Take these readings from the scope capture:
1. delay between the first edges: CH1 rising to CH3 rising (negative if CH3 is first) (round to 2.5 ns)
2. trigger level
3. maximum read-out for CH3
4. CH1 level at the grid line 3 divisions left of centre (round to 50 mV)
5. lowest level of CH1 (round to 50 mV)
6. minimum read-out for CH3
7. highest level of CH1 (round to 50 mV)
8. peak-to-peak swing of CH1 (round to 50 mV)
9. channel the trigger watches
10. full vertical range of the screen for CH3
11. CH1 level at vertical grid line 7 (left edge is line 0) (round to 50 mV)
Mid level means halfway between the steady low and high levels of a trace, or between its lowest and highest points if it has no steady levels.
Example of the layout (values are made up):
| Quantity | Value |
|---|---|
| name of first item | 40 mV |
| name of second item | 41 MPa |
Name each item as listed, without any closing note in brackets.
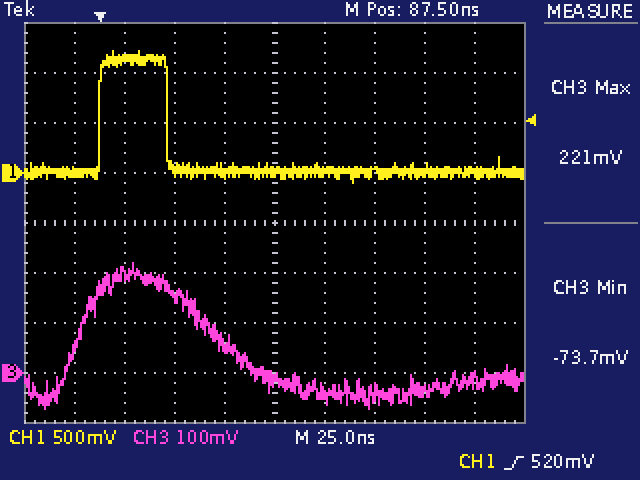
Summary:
| Quantity | Value |
|---|---|
| delay between the first edges: CH1 rising to CH3 rising (negative if CH3 is first) | -10.0 ns |
| trigger level | 520 mV |
| maximum read-out for CH3 | 221 mV |
| CH1 level at the grid line 3 divisions left of centre | 1.15 V |
| lowest level of CH1 | -100 mV |
| minimum read-out for CH3 | -73.7 mV |
| highest level of CH1 | 1.20 V |
| peak-to-peak swing of CH1 | 1.30 V |
| channel the trigger watches | CH1 |
| full vertical range of the screen for CH3 | 800 mV |
| CH1 level at vertical grid line 7 (left edge is line 0) | 0 mV |
